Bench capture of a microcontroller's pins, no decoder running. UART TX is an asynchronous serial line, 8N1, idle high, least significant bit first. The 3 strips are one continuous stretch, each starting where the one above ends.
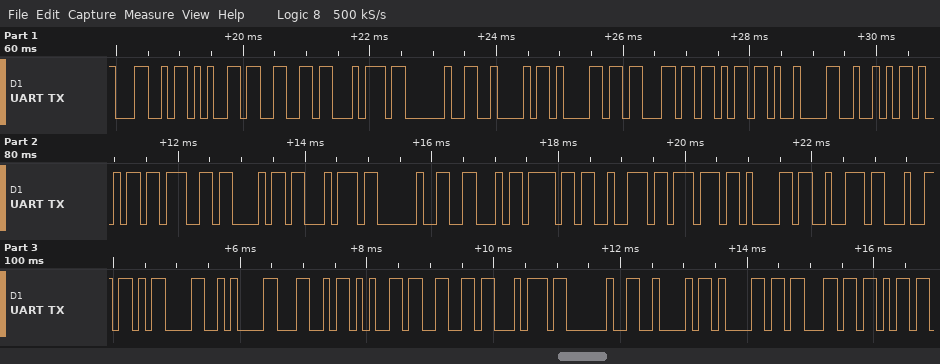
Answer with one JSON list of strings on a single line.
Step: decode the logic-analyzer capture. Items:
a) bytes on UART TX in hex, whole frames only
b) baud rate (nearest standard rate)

["0x4C 0x65 0x66 0x74 0x20 0x42 0x61 0x63 0x6B 0x09 0x52 0x69 0x67 0x68 0x74 0x20 0x46 0x6F 0x72 0x77 0x61 0x72 0x64 0x0D 0x0A 0x4C 0x65 0x66 0x74 0x20 0x42 0x61 0x63 0x6B", "9600 baud"]
